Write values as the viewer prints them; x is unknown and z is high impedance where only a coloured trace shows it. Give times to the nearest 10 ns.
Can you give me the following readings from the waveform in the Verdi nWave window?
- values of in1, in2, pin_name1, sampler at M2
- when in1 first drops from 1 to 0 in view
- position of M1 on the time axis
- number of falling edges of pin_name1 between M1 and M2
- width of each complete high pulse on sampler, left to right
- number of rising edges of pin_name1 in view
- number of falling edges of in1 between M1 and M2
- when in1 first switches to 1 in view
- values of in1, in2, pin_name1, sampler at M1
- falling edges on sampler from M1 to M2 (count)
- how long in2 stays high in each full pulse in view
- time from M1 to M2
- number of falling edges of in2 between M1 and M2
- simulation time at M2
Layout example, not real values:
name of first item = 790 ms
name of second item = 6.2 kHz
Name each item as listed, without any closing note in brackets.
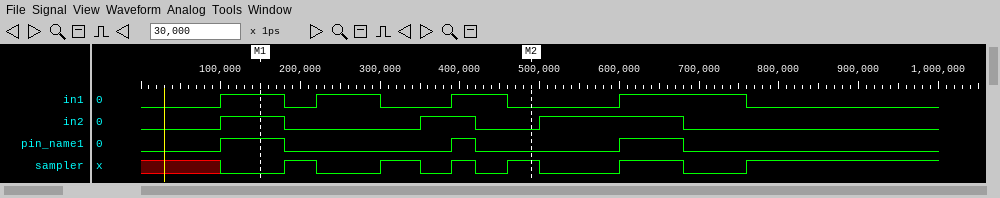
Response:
values of in1, in2, pin_name1, sampler at M2 = in1=0, in2=0, pin_name1=0, sampler=1
when in1 first drops from 1 to 0 in view = 180 ns
position of M1 on the time axis = 150 ns
number of falling edges of pin_name1 between M1 and M2 = 2
width of each complete high pulse on sampler, left to right = 40 ns, 50 ns, 30 ns, 40 ns, 80 ns
number of rising edges of pin_name1 in view = 3
number of falling edges of in1 between M1 and M2 = 3
when in1 first switches to 1 in view = 100 ns
values of in1, in2, pin_name1, sampler at M1 = in1=1, in2=1, pin_name1=1, sampler=0
falling edges on sampler from M1 to M2 = 3
how long in2 stays high in each full pulse in view = 80 ns, 70 ns, 180 ns
time from M1 to M2 = 340 ns
number of falling edges of in2 between M1 and M2 = 2
simulation time at M2 = 490 ns
